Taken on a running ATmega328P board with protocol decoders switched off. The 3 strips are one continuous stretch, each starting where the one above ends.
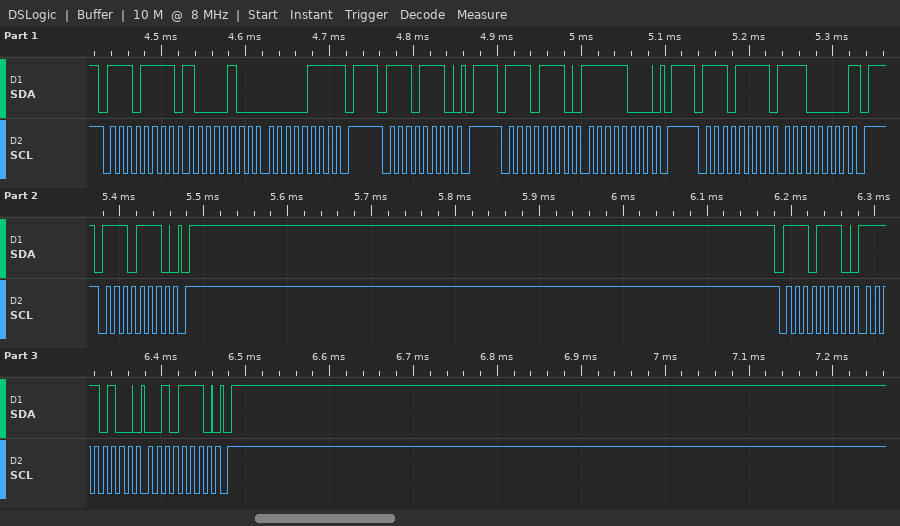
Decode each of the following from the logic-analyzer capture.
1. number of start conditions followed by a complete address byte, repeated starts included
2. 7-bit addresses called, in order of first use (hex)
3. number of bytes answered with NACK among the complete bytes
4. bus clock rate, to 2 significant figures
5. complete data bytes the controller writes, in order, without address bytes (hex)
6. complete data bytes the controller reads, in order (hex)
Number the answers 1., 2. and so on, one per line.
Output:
1. 6
2. 0x77
3. 2
4. 100 kHz
5. F8 F4 2E
6. 84 07 E0
